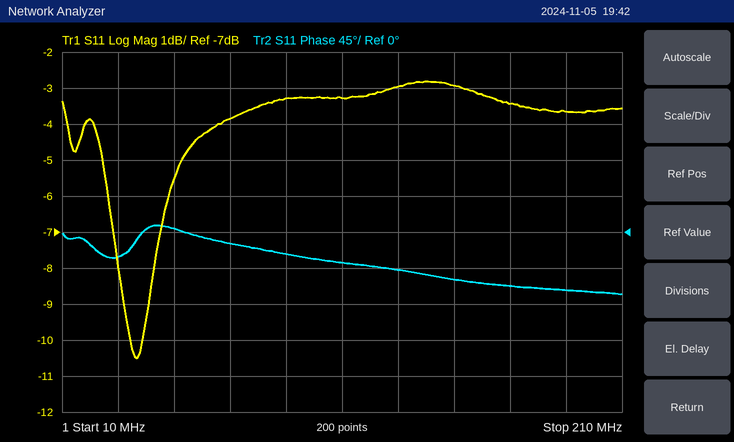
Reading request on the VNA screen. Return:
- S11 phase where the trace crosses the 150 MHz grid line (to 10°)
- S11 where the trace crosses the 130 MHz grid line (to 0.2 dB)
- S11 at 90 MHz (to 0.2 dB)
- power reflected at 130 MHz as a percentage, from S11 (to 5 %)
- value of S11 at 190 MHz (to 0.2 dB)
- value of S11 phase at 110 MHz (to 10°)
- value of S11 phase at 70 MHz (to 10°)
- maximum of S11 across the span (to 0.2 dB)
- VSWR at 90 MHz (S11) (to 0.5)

-60°
-3.0 dB
-3.2 dB
50 %
-3.6 dB
-40°
-10°
-2.8 dB
5.5
